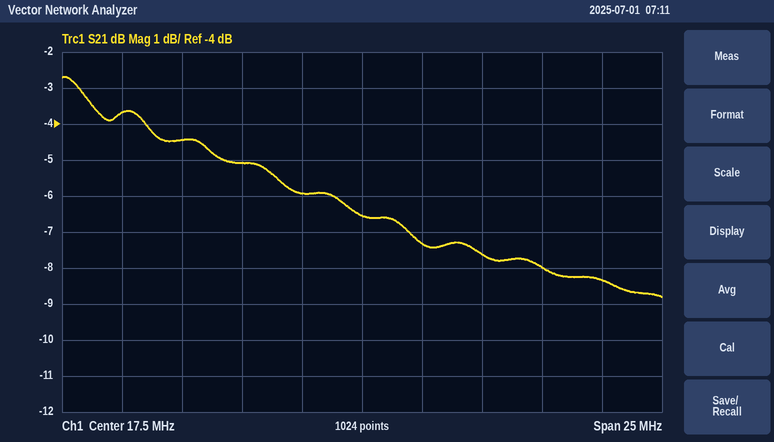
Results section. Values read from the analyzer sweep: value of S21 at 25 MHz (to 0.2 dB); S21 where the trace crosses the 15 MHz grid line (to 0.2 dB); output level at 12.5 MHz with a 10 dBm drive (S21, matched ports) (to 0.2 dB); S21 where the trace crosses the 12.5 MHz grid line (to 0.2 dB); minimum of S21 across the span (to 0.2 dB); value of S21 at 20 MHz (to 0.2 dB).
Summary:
-8.0 dB
-6.0 dB
5.0 dBm
-5.0 dB
-8.8 dB
-7.4 dB
